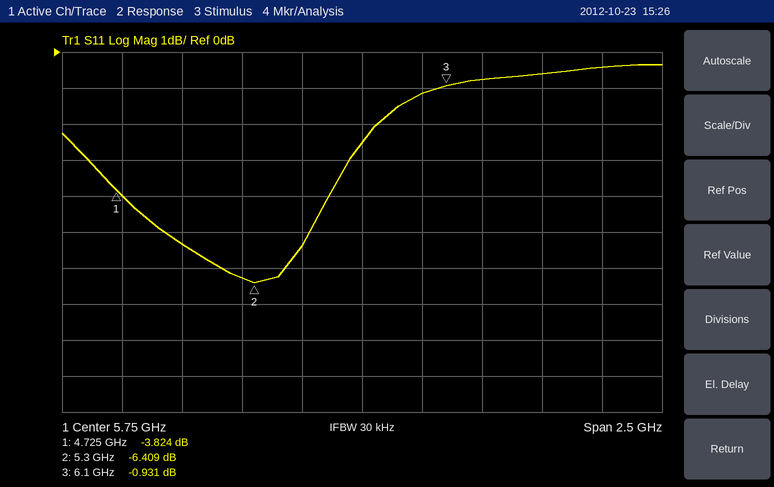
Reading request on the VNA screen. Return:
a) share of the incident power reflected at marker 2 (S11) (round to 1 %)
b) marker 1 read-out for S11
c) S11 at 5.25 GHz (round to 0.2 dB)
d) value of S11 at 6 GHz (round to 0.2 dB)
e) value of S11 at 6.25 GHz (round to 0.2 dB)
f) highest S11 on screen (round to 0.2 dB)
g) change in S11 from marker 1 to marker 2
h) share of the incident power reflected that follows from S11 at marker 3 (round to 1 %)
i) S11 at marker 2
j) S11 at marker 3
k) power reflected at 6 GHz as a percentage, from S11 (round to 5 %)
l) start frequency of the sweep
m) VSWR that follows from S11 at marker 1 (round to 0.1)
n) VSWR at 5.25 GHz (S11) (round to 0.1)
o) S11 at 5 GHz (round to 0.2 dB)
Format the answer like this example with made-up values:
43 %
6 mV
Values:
23 %
-3.824 dB
-6.2 dB
-1.2 dB
-0.8 dB
-0.4 dB
-2.585 dB
81 %
-6.409 dB
-0.931 dB
75 %
4.5 GHz
4.6
2.9
-5.4 dB
